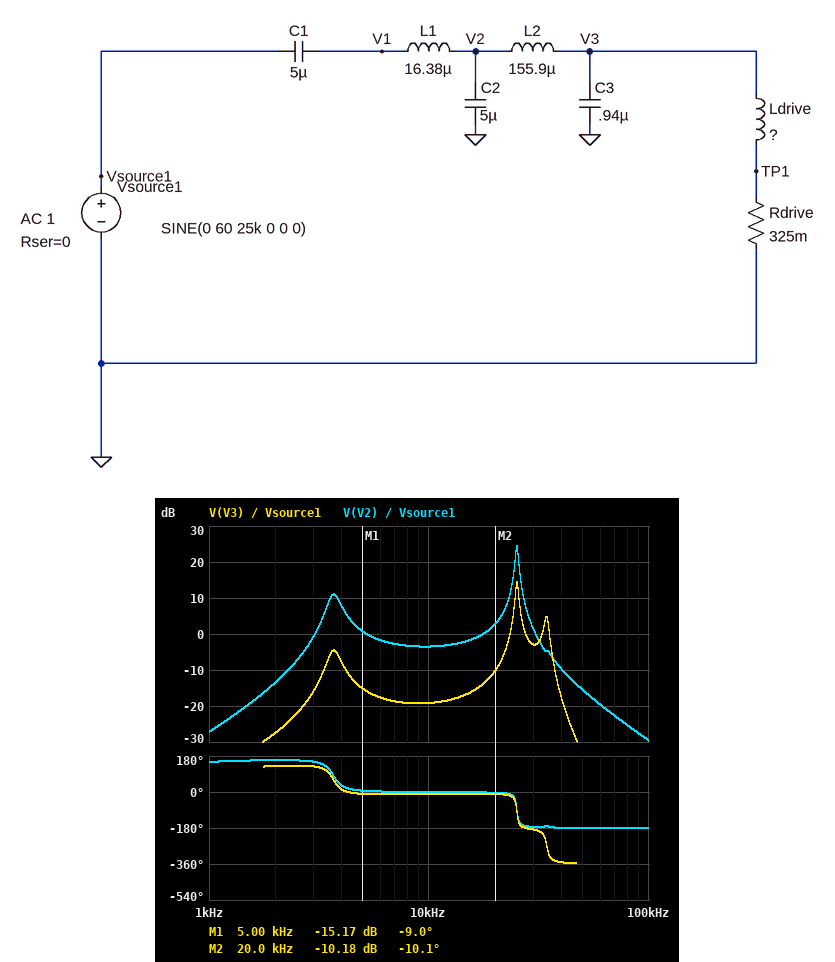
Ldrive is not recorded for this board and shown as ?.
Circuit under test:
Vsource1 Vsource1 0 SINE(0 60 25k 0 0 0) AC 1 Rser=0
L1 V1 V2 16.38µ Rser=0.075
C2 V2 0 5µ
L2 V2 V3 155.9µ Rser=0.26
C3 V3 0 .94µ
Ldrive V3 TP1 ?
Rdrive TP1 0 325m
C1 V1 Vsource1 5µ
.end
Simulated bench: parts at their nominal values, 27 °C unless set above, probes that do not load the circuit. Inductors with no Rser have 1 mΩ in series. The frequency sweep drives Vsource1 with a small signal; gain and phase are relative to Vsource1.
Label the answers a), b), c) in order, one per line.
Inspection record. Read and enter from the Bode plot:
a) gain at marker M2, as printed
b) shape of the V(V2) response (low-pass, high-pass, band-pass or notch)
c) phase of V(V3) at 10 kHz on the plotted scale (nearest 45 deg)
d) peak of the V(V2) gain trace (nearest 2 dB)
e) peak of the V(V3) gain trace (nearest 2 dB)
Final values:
a) -10.18 dB
b) band-pass
c) 0 deg
d) 24 dB
e) 14 dB
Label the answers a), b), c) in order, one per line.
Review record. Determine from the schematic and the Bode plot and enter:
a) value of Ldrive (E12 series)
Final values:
a) 27 µH
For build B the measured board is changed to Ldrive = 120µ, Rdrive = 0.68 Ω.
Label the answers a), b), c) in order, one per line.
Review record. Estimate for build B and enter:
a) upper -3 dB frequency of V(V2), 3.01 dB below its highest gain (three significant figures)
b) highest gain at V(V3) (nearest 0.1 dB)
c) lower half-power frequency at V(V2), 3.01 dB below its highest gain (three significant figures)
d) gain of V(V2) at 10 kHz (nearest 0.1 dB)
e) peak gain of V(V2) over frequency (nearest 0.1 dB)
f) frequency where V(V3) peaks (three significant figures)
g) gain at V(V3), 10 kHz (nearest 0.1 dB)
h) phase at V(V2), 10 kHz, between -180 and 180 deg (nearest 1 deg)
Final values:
a) 25.8 kHz
b) 24.5 dB
c) 25.1 kHz
d) -4.0 dB
e) 24.8 dB
f) 19.8 kHz
g) -8.7 dB
h) 0 deg
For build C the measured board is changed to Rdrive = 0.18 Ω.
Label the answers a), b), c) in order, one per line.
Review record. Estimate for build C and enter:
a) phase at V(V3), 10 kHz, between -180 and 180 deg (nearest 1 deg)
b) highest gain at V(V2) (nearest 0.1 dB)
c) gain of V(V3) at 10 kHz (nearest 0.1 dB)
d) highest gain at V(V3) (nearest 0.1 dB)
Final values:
a) -5 deg
b) 24.6 dB
c) -19.3 dB
d) 14.7 dB
